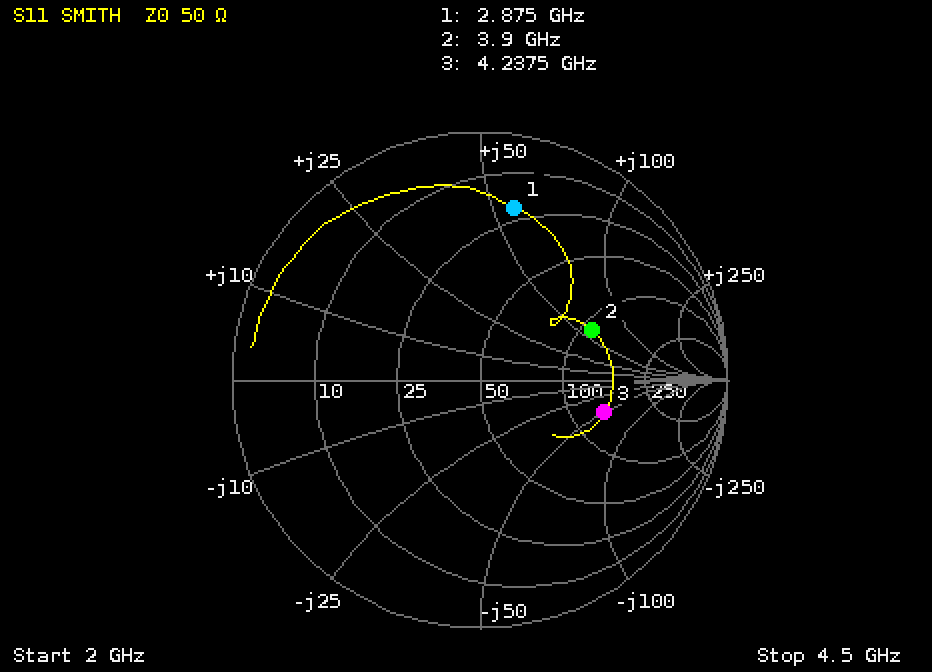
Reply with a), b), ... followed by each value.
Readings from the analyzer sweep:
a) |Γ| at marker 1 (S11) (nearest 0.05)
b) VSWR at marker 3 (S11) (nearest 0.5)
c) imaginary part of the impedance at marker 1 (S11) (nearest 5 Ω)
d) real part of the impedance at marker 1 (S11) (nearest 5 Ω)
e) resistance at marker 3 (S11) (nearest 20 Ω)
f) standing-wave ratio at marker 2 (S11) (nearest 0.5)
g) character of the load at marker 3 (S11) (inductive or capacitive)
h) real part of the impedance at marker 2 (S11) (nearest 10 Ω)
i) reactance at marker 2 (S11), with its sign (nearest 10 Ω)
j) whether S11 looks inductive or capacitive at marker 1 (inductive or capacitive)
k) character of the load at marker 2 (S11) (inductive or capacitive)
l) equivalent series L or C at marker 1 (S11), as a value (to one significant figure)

a) 0.70
b) 3.0
c) +55 Ω
d) 20 Ω
e) 140 Ω
f) 3.0
g) capacitive
h) 110 Ω
i) +60 Ω
j) inductive
k) inductive
l) 3 nH
